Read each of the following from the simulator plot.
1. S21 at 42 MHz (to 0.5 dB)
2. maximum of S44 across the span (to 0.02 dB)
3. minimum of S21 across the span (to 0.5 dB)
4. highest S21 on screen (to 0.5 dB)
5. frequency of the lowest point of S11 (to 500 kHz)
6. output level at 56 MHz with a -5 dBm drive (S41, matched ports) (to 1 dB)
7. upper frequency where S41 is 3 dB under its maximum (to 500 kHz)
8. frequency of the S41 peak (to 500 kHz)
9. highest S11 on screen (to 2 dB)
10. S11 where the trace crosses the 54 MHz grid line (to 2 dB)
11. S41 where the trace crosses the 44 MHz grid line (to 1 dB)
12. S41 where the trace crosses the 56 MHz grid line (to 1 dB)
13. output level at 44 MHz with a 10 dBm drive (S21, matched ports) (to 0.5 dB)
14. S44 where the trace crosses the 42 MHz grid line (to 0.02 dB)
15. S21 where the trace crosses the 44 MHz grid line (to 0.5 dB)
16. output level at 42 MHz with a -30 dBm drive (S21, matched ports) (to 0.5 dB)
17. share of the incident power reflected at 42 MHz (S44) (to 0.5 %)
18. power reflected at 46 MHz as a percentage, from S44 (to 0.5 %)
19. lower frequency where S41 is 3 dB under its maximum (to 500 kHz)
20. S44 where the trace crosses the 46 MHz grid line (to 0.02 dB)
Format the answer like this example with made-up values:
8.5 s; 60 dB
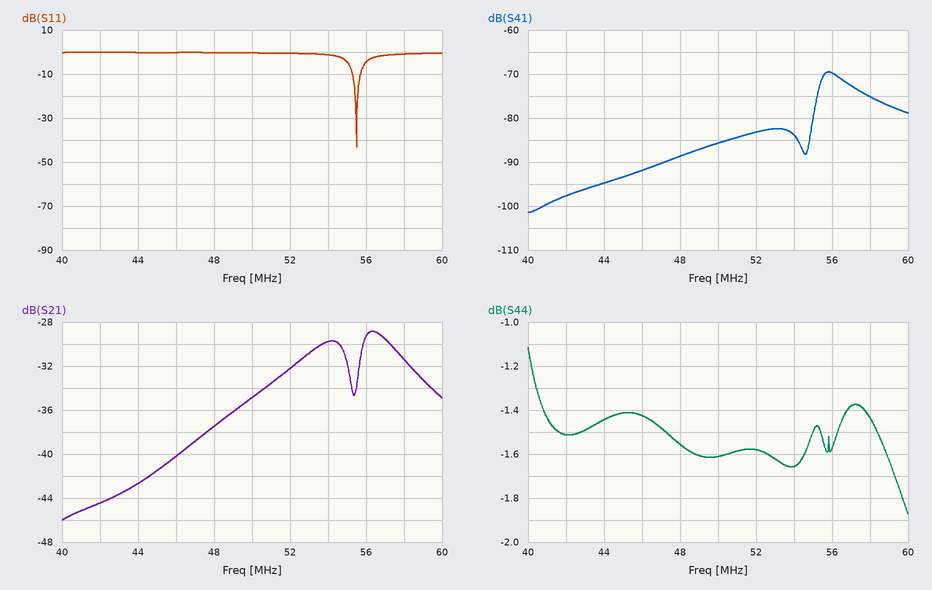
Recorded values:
-44.5 dB; -1.12 dB; -46.0 dB; -29.0 dB; 55.5 MHz; -75 dBm; 57.0 MHz; 56.0 MHz; 0 dB; -2 dB; -95 dB; -70 dB; -32.5 dBm; -1.52 dB; -42.5 dB; -74.5 dBm; 70.5 %; 72.0 %; 55.5 MHz; -1.42 dB
